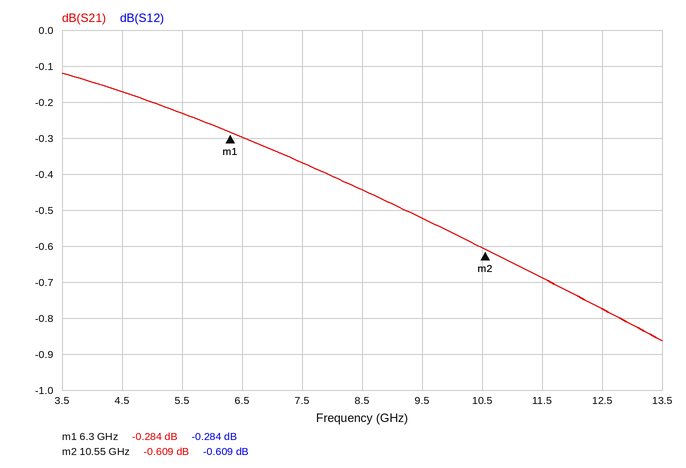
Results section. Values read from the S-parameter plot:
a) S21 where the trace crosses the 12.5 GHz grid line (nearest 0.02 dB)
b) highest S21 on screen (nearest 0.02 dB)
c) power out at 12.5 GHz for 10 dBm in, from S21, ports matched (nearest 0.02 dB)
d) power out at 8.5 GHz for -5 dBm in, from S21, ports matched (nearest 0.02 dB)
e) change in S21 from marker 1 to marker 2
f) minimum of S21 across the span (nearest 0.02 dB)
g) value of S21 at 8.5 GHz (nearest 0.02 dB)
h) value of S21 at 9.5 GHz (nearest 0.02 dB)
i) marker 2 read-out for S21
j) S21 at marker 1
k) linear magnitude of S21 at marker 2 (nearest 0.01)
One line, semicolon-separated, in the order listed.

-0.78 dB; -0.12 dB; 9.22 dBm; -5.44 dBm; -0.325 dB; -0.86 dB; -0.44 dB; -0.52 dB; -0.609 dB; -0.284 dB; 0.93
